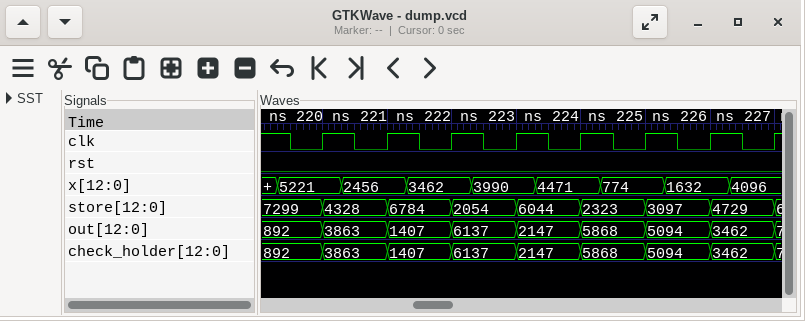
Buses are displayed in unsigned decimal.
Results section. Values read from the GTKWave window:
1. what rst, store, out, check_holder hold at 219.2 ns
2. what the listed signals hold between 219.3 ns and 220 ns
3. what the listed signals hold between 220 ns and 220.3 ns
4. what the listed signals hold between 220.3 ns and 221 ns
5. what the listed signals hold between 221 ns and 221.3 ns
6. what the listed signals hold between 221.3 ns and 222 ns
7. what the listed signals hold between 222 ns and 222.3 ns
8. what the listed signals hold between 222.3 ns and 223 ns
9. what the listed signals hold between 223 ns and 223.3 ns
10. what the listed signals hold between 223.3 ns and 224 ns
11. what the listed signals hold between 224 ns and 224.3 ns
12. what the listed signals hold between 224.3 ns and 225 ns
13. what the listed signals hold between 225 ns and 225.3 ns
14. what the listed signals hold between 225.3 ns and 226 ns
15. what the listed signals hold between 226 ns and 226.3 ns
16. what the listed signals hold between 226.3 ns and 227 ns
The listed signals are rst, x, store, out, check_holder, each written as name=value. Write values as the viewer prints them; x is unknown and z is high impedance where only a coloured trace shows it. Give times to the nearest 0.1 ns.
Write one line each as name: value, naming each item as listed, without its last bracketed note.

what rst, store, out, check_holder hold at 219.2 ns: rst=0, store=7299, out=892, check_holder=892
what the listed signals hold between 219.3 ns and 220 ns: rst=0, x=5221, store=7299, out=892, check_holder=892
what the listed signals hold between 220 ns and 220.3 ns: rst=0, x=5221, store=4328, out=3863, check_holder=3863
what the listed signals hold between 220.3 ns and 221 ns: rst=0, x=2456, store=4328, out=3863, check_holder=3863
what the listed signals hold between 221 ns and 221.3 ns: rst=0, x=2456, store=6784, out=1407, check_holder=1407
what the listed signals hold between 221.3 ns and 222 ns: rst=0, x=3462, store=6784, out=1407, check_holder=1407
what the listed signals hold between 222 ns and 222.3 ns: rst=0, x=3462, store=2054, out=6137, check_holder=6137
what the listed signals hold between 222.3 ns and 223 ns: rst=0, x=3990, store=2054, out=6137, check_holder=6137
what the listed signals hold between 223 ns and 223.3 ns: rst=0, x=3990, store=6044, out=2147, check_holder=2147
what the listed signals hold between 223.3 ns and 224 ns: rst=0, x=4471, store=6044, out=2147, check_holder=2147
what the listed signals hold between 224 ns and 224.3 ns: rst=0, x=4471, store=2323, out=5868, check_holder=5868
what the listed signals hold between 224.3 ns and 225 ns: rst=0, x=774, store=2323, out=5868, check_holder=5868
what the listed signals hold between 225 ns and 225.3 ns: rst=0, x=774, store=3097, out=5094, check_holder=5094
what the listed signals hold between 225.3 ns and 226 ns: rst=0, x=1632, store=3097, out=5094, check_holder=5094
what the listed signals hold between 226 ns and 226.3 ns: rst=0, x=1632, store=4729, out=3462, check_holder=3462
what the listed signals hold between 226.3 ns and 227 ns: rst=0, x=4096, store=4729, out=3462, check_holder=3462
